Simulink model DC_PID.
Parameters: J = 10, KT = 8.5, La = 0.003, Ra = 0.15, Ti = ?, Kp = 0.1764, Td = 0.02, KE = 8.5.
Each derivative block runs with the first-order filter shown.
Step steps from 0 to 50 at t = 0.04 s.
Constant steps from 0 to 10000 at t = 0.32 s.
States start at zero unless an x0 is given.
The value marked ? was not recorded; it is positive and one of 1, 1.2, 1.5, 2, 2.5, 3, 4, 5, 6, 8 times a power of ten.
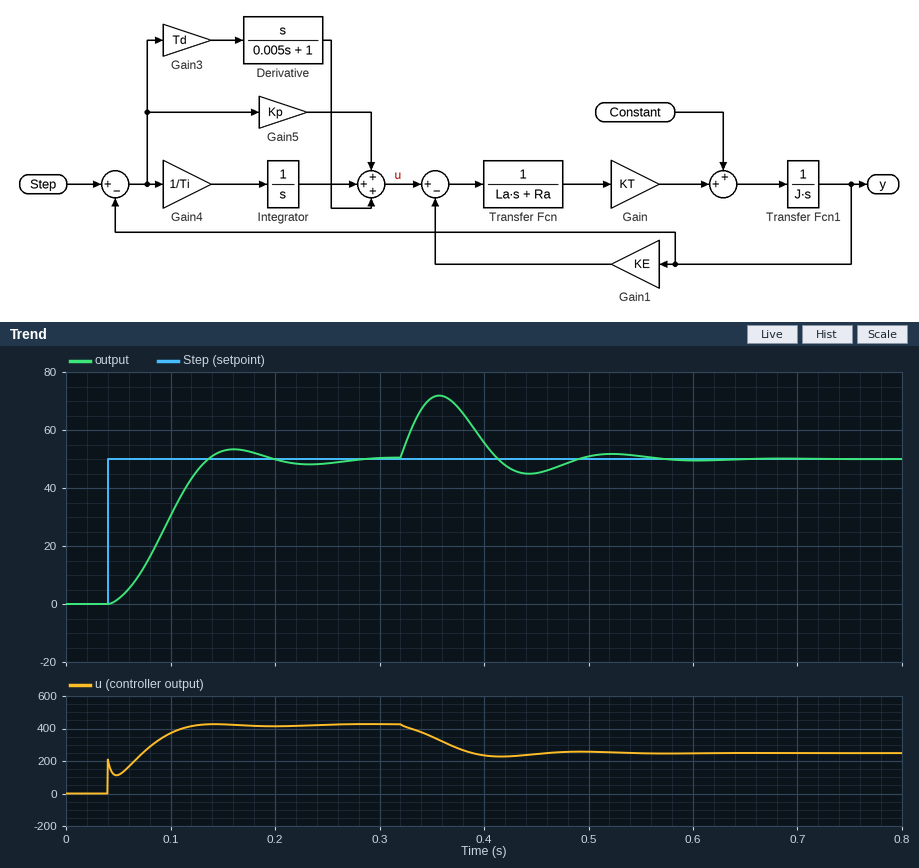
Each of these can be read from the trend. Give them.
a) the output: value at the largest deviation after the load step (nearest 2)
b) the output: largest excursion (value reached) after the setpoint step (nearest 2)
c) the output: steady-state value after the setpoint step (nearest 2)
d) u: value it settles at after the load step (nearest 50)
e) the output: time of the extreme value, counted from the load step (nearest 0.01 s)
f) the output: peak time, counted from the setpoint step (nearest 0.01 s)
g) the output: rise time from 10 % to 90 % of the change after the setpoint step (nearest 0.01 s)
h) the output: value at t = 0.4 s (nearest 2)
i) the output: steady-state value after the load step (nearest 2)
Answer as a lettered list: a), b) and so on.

a) 72
b) 54
c) 50
d) 250
e) 0.04 s
f) 0.12 s
g) 0.06 s
h) 56
i) 50
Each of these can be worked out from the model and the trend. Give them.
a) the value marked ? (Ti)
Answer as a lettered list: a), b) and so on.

a) 0.006
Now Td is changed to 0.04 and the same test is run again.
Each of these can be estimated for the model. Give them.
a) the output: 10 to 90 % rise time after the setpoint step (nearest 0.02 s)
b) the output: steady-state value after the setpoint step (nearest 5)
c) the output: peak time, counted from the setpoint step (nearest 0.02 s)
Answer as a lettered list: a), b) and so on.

a) 0.08 s
b) 50
c) 0.14 s
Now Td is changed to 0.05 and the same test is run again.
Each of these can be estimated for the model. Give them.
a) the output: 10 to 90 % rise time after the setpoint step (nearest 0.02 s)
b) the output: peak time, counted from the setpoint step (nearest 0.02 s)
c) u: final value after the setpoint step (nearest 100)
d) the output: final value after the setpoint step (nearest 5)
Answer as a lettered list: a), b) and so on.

a) 0.08 s
b) 0.14 s
c) 400
d) 50
